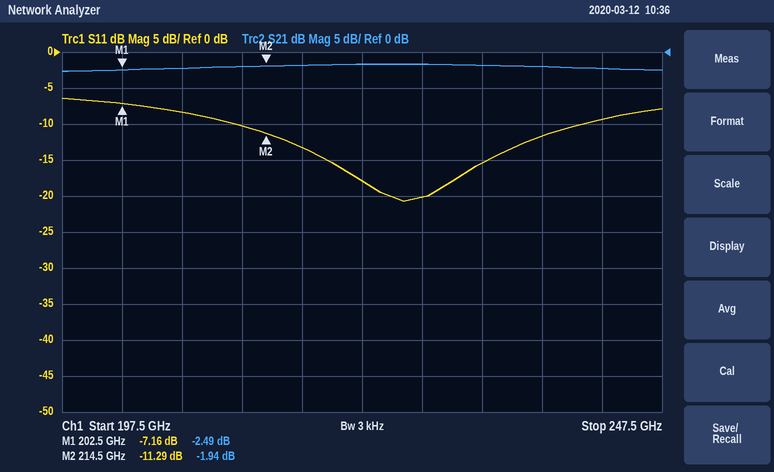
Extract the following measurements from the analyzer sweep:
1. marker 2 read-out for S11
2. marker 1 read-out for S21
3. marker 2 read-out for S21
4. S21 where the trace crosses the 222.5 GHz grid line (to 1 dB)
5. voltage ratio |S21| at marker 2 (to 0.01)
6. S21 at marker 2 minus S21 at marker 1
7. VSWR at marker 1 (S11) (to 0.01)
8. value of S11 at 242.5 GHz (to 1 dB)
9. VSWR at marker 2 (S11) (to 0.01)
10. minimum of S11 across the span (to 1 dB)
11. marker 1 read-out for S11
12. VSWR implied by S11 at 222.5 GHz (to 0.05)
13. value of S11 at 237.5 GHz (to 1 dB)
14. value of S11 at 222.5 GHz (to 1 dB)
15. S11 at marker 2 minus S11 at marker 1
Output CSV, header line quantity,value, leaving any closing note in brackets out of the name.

quantity,value
marker 2 read-out for S11,-11.29 dB
marker 1 read-out for S21,-2.49 dB
marker 2 read-out for S21,-1.94 dB
S21 where the trace crosses the 222.5 GHz grid line,-2 dB
voltage ratio |S21| at marker 2,0.80
S21 at marker 2 minus S21 at marker 1,0.55 dB
VSWR at marker 1 (S11),2.56
value of S11 at 242.5 GHz,-9 dB
VSWR at marker 2 (S11),1.75
minimum of S11 across the span,-21 dB
marker 1 read-out for S11,-7.16 dB
VSWR implied by S11 at 222.5 GHz,1.30
value of S11 at 237.5 GHz,-12 dB
value of S11 at 222.5 GHz,-18 dB
S11 at marker 2 minus S11 at marker 1,-4.13 dB
